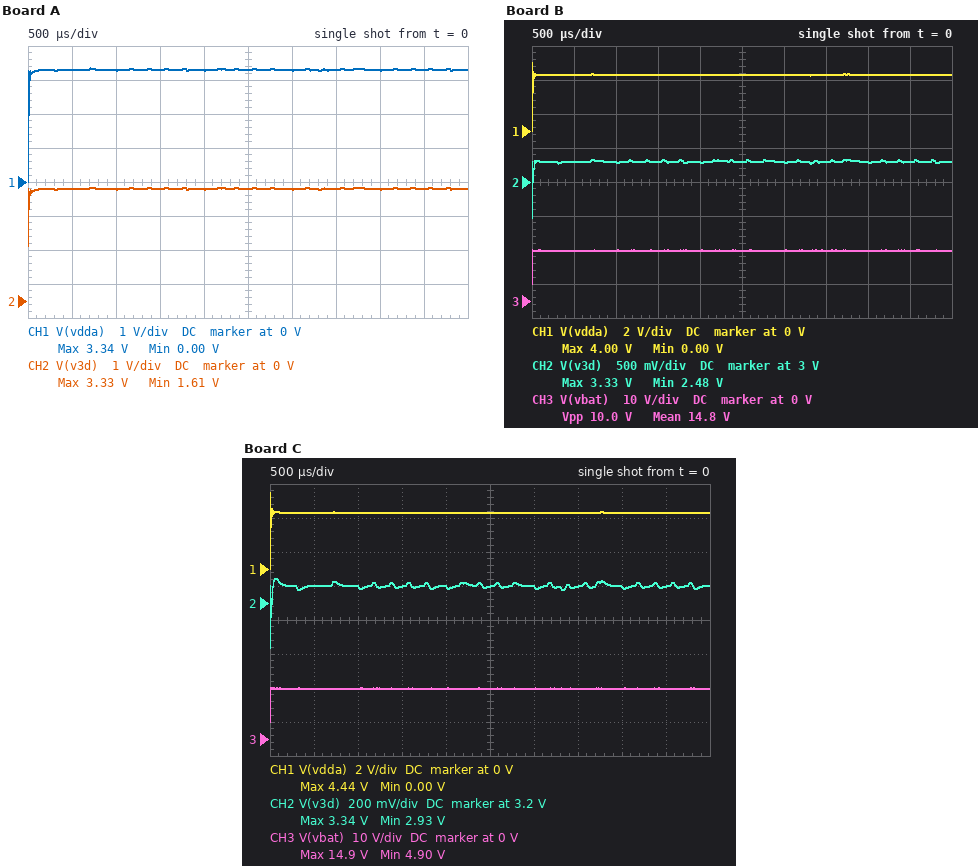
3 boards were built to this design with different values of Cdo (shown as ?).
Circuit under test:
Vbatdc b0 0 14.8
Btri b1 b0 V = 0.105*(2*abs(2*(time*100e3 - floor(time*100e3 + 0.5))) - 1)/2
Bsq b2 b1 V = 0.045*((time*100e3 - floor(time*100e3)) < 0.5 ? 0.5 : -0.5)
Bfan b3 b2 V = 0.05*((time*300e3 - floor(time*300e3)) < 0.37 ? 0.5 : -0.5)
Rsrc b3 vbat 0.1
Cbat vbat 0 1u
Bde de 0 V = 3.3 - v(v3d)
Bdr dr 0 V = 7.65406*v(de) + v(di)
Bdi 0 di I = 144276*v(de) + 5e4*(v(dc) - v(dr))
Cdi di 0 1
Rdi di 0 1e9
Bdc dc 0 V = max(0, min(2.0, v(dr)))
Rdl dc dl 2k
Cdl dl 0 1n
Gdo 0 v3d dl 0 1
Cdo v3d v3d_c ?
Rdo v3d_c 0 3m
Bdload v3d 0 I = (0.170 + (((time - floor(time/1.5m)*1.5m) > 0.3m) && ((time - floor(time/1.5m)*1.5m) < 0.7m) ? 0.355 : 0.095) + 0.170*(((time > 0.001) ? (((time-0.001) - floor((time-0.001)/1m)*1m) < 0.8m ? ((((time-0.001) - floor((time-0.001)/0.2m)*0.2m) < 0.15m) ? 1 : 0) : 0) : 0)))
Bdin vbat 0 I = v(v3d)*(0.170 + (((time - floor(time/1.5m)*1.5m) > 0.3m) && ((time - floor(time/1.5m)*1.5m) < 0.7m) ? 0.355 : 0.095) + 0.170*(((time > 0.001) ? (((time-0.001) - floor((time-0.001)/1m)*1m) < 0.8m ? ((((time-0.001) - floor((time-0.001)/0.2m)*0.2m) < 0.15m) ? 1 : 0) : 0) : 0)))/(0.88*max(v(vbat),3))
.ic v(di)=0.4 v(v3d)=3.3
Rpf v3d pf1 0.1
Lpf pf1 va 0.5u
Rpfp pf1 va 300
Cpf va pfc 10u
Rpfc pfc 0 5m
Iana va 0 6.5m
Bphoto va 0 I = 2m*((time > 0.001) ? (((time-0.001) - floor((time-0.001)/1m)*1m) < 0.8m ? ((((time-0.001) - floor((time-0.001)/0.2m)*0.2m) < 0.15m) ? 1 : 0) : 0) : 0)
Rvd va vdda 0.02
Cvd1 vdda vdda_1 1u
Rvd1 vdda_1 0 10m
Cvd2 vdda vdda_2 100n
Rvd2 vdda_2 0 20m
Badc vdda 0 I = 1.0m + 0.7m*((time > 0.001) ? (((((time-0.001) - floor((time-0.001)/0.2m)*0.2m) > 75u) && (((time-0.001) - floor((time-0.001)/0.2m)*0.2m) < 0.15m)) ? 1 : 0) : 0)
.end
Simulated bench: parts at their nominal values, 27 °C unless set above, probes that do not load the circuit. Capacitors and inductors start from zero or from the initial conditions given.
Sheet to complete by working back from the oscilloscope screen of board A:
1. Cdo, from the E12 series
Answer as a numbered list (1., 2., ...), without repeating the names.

1. 18 µF
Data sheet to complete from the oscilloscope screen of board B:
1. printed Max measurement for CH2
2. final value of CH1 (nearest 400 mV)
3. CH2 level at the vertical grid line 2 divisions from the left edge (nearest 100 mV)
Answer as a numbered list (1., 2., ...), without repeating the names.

1. 3.33 V
2. 3.2 V
3. 3.3 V
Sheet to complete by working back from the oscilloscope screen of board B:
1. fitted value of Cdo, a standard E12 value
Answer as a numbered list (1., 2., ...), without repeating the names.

1. 47 µF
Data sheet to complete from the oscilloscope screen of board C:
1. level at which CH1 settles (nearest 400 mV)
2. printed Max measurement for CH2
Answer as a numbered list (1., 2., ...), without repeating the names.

1. 3.2 V
2. 3.34 V
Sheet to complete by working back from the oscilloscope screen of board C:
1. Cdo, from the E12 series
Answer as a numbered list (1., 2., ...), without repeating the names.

1. 120 µF
